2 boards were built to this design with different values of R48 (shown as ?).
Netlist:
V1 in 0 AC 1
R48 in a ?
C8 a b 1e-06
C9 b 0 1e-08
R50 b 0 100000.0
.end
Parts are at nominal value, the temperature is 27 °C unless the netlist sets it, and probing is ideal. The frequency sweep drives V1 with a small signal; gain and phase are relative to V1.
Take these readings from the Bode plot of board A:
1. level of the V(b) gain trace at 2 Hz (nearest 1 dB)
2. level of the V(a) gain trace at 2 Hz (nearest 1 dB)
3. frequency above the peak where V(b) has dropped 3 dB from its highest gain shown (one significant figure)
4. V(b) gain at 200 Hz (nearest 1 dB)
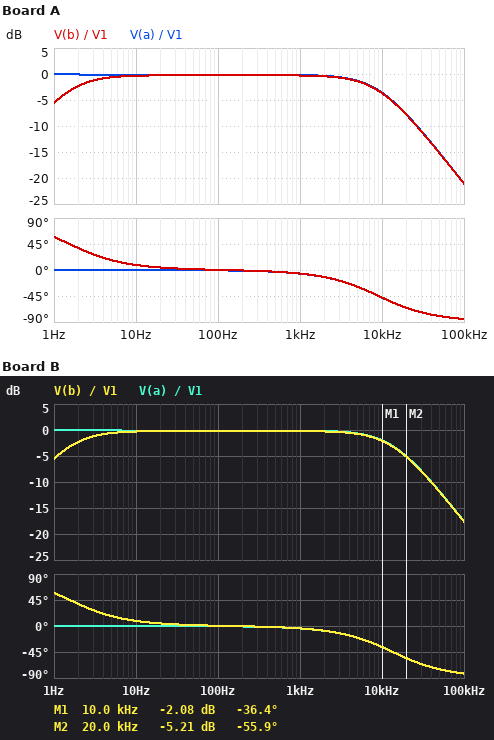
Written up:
-2 dB
0 dB
9 kHz
0 dB
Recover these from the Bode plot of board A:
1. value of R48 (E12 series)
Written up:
1.8 kΩ
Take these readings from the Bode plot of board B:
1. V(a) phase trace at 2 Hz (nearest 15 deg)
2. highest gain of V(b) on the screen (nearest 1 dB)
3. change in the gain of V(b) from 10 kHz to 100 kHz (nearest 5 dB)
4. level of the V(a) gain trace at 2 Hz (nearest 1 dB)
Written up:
0 deg
0 dB
-15 dB
0 dB
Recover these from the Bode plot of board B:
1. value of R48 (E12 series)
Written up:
1.2 kΩ
